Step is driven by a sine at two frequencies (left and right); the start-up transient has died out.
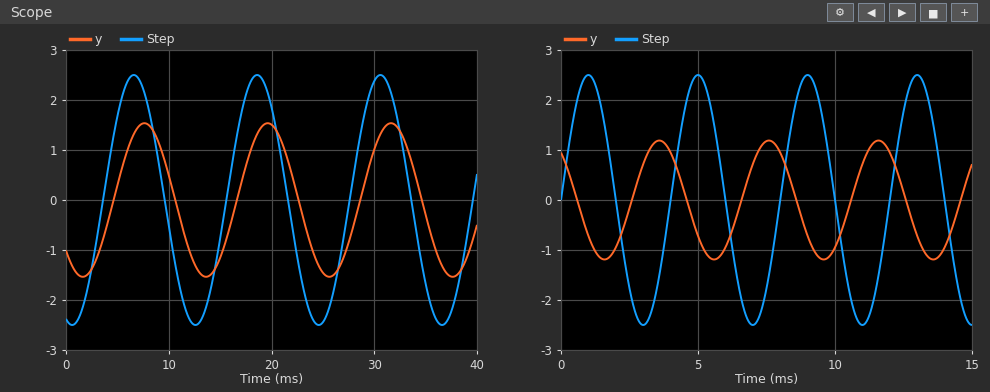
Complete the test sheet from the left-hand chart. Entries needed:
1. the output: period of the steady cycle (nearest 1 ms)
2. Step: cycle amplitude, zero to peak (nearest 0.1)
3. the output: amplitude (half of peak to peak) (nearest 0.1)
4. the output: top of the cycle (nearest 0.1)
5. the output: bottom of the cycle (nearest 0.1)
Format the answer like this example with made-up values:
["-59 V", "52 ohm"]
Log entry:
["12 ms", "2.5", "1.5", "1.5", "-1.5"]
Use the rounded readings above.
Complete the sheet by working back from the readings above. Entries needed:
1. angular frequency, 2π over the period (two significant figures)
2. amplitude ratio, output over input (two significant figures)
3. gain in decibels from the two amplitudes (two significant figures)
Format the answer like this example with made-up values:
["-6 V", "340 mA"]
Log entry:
["0.52 rad/ms", "0.60", "-4.4 dB"]
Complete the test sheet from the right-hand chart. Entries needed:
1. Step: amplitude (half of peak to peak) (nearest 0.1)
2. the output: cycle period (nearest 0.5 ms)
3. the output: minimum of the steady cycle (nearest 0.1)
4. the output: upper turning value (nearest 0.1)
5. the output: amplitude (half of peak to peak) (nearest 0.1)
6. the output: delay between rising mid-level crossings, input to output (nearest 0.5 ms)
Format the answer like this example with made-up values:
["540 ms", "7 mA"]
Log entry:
["2.5", "4.0 ms", "-1.2", "1.2", "1.2", "2.5 ms"]
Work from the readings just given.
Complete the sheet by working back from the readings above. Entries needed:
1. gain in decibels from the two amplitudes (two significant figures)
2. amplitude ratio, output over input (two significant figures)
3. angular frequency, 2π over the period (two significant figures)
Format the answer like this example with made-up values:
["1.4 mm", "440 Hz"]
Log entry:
["-6.4 dB", "0.48", "1.6 rad/ms"]
